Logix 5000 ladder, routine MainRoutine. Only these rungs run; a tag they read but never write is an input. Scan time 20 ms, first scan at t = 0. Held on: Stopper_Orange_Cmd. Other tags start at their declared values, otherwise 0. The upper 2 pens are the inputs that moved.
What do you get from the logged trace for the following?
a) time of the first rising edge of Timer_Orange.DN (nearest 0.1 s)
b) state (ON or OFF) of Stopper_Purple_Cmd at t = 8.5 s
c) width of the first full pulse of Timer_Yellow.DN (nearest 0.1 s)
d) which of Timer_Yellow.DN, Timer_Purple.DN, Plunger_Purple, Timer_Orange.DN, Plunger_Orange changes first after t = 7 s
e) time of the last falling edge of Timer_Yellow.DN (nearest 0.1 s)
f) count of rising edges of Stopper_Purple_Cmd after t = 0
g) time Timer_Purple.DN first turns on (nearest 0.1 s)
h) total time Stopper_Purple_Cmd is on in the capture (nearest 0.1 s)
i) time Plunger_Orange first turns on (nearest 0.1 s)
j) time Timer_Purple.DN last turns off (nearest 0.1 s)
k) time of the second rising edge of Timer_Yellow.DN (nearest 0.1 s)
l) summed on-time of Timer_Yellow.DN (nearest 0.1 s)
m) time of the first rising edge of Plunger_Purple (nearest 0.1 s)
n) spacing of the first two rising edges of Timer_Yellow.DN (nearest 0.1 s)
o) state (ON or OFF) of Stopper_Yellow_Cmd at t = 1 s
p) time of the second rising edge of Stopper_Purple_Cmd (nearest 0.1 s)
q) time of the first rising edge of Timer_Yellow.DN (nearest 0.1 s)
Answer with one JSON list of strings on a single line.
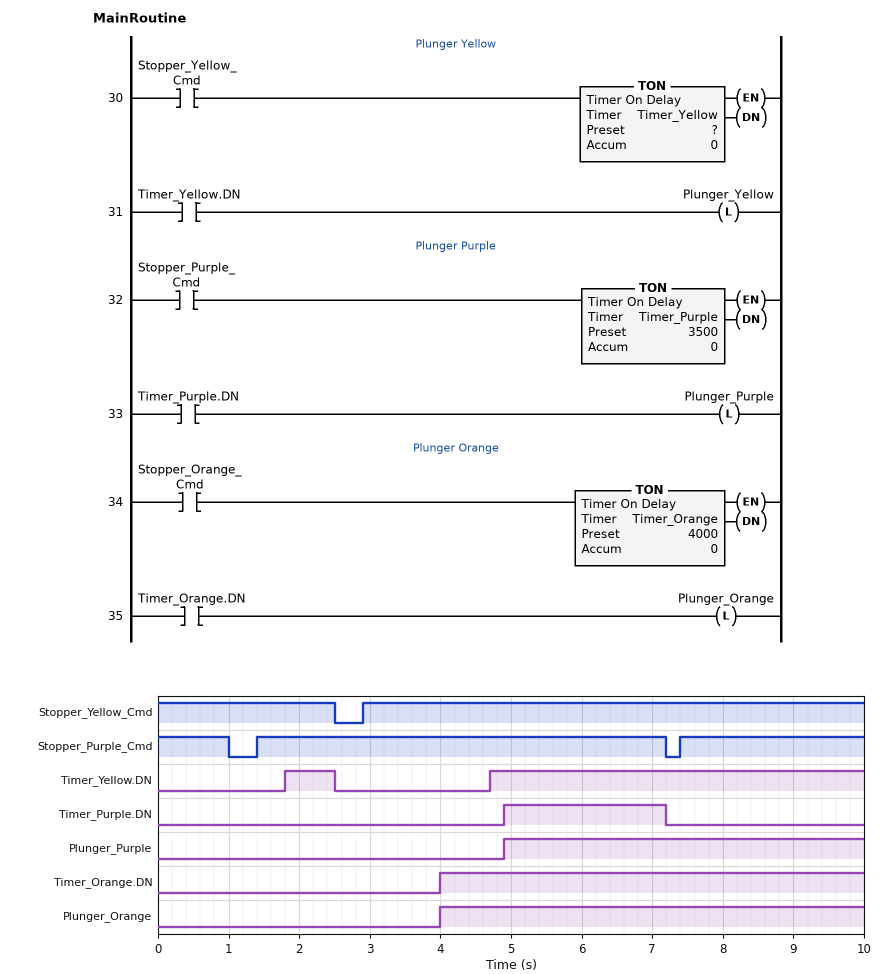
["4.0 s", "ON", "0.7 s", "Timer_Purple.DN", "2.5 s", "2", "4.9 s", "9.4 s", "4.0 s", "7.2 s", "4.7 s", "6.0 s", "4.9 s", "2.9 s", "ON", "7.4 s", "1.8 s"]
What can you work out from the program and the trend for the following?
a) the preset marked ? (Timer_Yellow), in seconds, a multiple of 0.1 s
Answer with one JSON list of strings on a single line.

["1.8 s"]
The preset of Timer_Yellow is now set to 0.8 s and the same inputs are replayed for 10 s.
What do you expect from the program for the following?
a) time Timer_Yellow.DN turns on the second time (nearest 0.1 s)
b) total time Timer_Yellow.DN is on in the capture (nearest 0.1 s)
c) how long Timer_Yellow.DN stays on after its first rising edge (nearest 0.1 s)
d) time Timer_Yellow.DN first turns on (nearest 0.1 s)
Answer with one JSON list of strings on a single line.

["3.7 s", "8.0 s", "1.7 s", "0.8 s"]
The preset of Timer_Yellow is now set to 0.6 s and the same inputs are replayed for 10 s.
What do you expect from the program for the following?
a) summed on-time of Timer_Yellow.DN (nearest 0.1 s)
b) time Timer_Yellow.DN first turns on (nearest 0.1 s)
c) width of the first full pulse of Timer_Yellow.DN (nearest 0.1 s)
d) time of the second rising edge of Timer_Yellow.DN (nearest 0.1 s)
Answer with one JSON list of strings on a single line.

["8.4 s", "0.6 s", "1.9 s", "3.5 s"]
